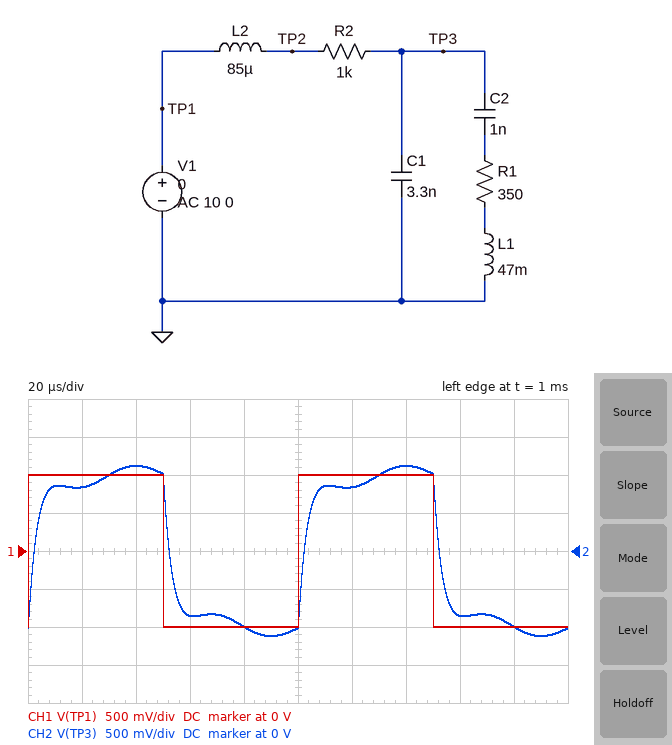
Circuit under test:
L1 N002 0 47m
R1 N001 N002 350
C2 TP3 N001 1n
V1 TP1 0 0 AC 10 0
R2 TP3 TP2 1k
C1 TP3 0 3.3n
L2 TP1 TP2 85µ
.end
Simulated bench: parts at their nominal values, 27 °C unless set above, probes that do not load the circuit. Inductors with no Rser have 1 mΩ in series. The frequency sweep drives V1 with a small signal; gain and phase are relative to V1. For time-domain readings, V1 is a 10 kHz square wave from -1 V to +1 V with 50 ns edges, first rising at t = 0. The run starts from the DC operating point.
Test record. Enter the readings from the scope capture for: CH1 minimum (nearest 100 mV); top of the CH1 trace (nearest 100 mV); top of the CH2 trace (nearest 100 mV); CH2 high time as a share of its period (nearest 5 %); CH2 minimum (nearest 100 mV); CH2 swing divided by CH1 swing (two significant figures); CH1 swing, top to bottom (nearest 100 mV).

-1.0 V
1.0 V
1.1 V
50 %
-1.1 V
1.1
2.0 V
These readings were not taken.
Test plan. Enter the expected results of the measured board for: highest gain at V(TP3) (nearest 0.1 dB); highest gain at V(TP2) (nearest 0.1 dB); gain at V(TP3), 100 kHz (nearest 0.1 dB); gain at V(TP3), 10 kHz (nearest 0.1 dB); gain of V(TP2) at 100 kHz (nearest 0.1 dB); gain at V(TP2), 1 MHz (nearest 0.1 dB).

0 dB
0.2 dB
-6.9 dB
-0.3 dB
0.2 dB
-0.9 dB
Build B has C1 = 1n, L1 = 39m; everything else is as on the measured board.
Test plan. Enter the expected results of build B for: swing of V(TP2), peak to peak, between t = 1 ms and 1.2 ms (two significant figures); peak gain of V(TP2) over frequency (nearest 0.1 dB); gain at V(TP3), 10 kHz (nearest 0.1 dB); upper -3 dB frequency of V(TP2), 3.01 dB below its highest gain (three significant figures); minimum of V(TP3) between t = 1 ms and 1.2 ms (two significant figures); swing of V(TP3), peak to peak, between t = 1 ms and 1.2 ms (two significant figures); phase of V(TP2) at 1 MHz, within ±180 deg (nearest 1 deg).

2.3 V
0.5 dB
-0.1 dB
1.82 MHz
-1.2 V
2.4 V
-30 deg
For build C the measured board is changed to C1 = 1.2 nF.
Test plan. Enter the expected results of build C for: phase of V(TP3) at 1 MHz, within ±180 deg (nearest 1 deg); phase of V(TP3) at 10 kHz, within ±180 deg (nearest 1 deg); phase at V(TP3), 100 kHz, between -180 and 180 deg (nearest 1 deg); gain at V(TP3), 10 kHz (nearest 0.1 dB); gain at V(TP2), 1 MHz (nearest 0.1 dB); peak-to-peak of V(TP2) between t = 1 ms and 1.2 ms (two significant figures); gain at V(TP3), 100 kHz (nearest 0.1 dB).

-112 deg
-9 deg
-37 deg
-0.1 dB
-0.6 dB
2.2 V
-1.6 dB
